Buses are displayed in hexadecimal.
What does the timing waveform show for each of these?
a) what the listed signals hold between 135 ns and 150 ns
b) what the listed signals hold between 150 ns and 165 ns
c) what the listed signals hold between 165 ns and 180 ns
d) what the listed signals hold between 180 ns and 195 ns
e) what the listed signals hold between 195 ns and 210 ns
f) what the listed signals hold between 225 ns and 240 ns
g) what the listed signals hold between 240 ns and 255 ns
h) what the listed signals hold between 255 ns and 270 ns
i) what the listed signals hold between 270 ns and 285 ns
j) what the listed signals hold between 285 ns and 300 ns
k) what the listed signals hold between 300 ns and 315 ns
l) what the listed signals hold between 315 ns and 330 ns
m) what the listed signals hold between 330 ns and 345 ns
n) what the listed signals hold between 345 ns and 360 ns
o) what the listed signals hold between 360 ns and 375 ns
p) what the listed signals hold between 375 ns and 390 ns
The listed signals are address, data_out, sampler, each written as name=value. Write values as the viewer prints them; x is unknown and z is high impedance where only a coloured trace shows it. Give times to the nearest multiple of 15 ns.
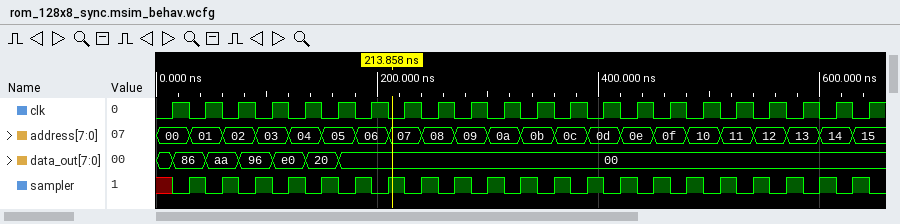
address=04, data_out=20, sampler=0
address=05, data_out=20, sampler=1
address=05, data_out=00, sampler=0
address=06, data_out=00, sampler=1
address=06, data_out=00, sampler=0
address=07, data_out=00, sampler=0
address=08, data_out=00, sampler=1
address=08, data_out=00, sampler=0
address=09, data_out=00, sampler=1
address=09, data_out=00, sampler=0
address=0a, data_out=00, sampler=1
address=0a, data_out=00, sampler=0
address=0b, data_out=00, sampler=1
address=0b, data_out=00, sampler=0
address=0c, data_out=00, sampler=1
address=0c, data_out=00, sampler=0
